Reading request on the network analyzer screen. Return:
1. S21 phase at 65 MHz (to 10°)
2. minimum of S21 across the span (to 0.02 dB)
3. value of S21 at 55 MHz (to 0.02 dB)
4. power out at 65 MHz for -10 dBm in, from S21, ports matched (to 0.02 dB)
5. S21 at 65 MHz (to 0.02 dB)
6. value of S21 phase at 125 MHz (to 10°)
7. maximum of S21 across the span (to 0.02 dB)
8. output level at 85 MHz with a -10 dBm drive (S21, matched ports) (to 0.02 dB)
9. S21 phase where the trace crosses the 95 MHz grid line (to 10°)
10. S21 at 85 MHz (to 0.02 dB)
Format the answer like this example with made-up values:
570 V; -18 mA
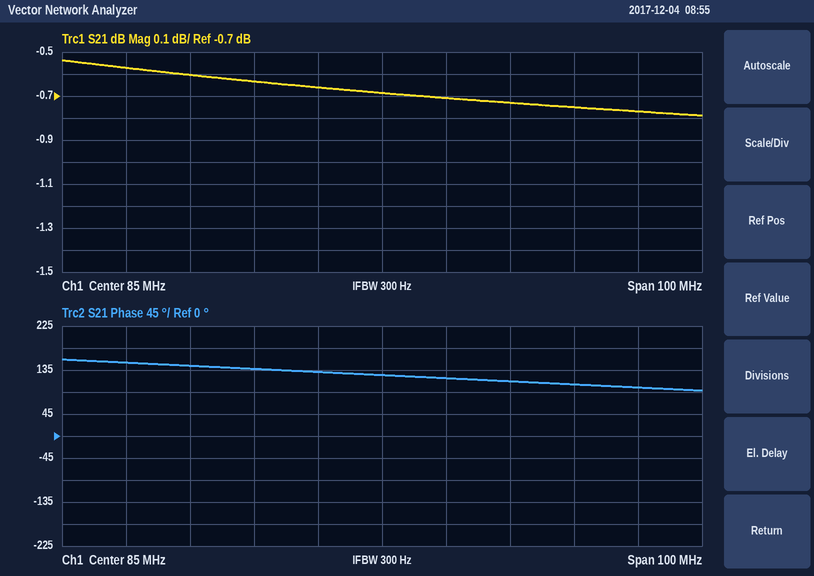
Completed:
140°; -0.78 dB; -0.60 dB; -10.64 dBm; -0.64 dB; 100°; -0.54 dB; -10.68 dBm; 120°; -0.68 dB
